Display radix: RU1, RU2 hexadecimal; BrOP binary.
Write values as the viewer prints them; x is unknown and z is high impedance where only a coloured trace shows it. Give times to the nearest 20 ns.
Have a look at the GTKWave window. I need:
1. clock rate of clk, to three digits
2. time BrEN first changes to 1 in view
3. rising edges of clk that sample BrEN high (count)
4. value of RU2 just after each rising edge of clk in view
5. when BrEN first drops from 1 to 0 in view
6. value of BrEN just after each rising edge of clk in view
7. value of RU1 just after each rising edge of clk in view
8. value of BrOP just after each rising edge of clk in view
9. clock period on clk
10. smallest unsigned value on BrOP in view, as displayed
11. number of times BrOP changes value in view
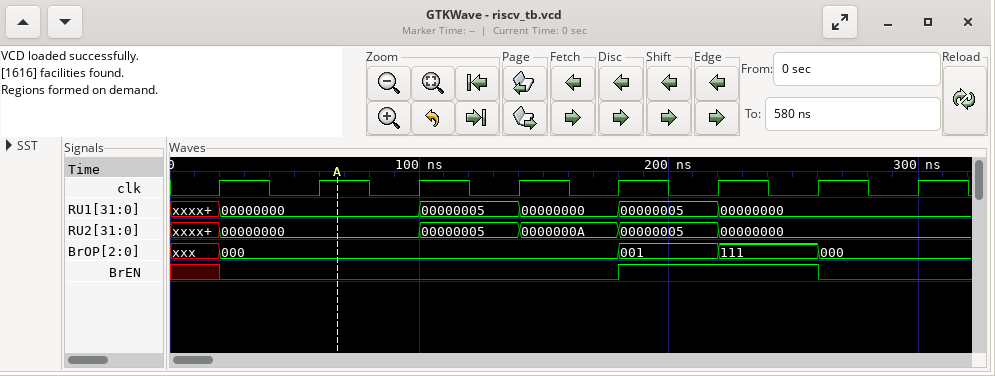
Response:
25.0 MHz
180 ns
2
00000000, 00000000, 00000005, 0000000A, 00000005, 00000000, 00000000, 00000000
260 ns
0 0 0 0 1 1 0 0
00000000, 00000000, 00000005, 00000000, 00000005, 00000000, 00000000, 00000000
000, 000, 000, 000, 001, 111, 000, 000
40 ns
000
4
